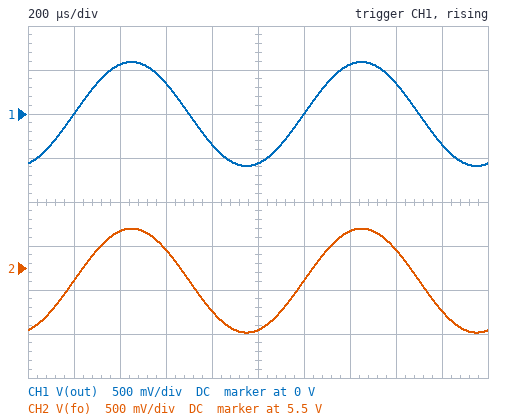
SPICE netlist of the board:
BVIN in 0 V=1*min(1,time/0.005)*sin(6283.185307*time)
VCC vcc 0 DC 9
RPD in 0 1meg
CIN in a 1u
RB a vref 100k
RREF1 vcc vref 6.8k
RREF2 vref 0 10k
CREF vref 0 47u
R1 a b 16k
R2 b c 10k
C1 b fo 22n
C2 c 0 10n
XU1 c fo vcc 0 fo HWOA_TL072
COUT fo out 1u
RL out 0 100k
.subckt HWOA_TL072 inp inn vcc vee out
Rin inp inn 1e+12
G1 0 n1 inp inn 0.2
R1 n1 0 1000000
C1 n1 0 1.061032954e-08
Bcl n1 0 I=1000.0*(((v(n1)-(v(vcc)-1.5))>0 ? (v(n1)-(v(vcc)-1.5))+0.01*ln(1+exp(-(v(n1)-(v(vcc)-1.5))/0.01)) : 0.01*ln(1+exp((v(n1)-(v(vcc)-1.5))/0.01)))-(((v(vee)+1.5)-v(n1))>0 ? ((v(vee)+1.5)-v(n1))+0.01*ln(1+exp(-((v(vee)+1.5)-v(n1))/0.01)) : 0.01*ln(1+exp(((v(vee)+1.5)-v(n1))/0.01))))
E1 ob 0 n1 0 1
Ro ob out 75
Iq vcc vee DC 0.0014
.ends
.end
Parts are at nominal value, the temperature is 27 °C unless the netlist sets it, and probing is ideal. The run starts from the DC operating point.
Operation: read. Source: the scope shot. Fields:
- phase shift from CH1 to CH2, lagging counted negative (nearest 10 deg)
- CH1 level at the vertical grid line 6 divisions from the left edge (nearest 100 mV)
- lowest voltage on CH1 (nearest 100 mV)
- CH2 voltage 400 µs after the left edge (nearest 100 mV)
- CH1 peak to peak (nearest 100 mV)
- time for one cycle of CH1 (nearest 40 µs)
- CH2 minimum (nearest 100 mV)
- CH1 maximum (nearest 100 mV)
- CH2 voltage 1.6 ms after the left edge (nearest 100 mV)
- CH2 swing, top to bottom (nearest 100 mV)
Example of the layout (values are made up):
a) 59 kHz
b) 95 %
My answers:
a) 0 deg
b) 0 V
c) -600 mV
d) 5.9 V
e) 1.2 V
f) 1.00 ms
g) 4.8 V
h) 600 mV
i) 5.7 V
j) 1.2 V
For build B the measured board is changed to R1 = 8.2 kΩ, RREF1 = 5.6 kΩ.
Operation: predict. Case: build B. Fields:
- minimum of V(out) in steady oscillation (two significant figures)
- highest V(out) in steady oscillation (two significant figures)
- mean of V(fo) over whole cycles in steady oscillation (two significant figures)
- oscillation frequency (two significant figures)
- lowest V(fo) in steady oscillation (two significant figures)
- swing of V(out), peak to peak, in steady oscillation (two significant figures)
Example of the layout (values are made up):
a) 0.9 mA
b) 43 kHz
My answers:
a) -840 mV
b) 840 mV
c) 5.8 V
d) 1.0 kHz
e) 4.9 V
f) 1.7 V
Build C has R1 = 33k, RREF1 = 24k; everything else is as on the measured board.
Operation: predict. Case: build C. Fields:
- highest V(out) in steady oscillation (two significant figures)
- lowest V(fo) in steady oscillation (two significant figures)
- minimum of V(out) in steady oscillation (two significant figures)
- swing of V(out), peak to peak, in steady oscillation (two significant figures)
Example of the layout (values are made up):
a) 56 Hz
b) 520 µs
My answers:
a) 300 mV
b) 2.3 V
c) -300 mV
d) 610 mV
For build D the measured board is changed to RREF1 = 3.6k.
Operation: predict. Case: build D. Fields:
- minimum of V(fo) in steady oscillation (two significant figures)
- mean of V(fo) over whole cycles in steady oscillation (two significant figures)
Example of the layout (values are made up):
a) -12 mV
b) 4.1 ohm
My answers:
a) 6.0 V
b) 6.6 V
